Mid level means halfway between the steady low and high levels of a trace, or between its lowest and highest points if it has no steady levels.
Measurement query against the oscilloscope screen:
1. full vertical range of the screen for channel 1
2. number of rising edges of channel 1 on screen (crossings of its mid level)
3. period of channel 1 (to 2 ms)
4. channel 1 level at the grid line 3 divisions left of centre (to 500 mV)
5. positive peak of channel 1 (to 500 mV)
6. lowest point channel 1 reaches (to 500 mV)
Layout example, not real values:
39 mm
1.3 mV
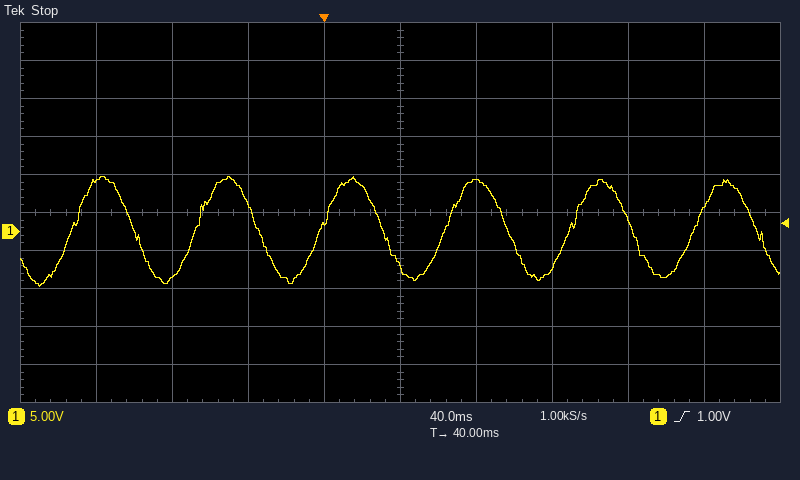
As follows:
50 V
6
66 ms
-6.0 V
7.0 V
-7.0 V
